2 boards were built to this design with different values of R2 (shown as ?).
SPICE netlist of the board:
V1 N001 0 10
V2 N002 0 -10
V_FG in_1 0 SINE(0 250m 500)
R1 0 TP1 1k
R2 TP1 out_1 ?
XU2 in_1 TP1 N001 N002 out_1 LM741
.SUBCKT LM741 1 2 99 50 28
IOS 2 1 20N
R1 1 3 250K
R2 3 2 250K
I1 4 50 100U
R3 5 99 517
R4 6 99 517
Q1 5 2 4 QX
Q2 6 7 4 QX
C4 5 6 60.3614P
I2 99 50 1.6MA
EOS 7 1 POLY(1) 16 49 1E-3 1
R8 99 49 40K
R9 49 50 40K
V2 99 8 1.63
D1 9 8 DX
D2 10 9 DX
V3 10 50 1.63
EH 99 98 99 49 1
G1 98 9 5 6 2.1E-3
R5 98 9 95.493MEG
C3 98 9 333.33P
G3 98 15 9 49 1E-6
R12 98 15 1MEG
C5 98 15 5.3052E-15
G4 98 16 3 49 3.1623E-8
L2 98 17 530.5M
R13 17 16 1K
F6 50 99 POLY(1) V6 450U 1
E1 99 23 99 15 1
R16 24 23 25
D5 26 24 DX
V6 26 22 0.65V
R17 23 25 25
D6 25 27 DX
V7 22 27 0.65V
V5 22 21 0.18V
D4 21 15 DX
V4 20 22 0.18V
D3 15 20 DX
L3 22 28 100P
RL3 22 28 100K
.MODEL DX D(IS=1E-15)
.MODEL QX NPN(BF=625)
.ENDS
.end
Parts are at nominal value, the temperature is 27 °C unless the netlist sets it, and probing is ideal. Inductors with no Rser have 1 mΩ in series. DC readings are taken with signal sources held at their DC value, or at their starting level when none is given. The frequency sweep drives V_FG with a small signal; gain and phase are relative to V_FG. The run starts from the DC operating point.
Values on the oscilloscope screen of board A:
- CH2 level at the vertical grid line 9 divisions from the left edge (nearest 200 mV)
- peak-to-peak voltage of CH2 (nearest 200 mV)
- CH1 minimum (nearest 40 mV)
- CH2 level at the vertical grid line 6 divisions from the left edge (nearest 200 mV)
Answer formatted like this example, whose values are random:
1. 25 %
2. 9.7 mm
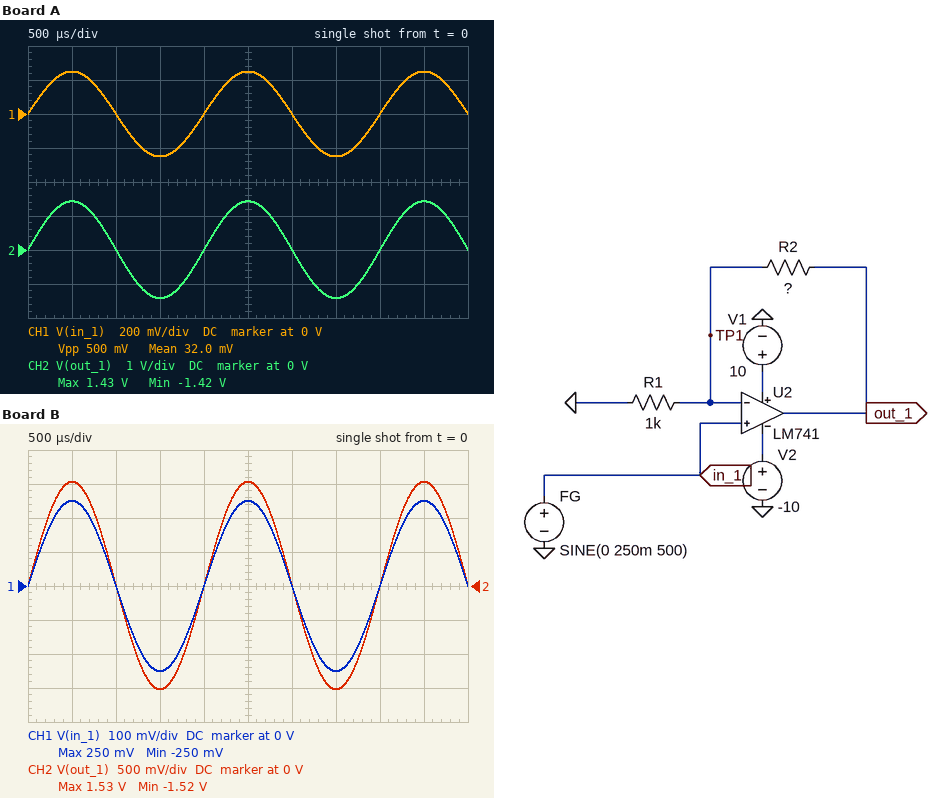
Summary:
1. 1.4 V
2. 2.8 V
3. -240 mV
4. 0 V
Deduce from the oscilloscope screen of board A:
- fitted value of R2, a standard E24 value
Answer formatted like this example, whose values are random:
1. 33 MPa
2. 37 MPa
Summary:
1. 4.7 kΩ
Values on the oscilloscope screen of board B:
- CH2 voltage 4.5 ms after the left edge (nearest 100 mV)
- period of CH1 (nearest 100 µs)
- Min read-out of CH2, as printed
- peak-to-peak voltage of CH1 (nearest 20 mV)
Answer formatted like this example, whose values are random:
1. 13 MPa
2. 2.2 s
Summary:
1. 1.5 V
2. 2.0 ms
3. -1.52 V
4. 500 mV
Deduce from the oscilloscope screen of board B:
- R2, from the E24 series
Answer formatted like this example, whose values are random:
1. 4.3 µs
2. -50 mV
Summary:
1. 5.1 kΩ
